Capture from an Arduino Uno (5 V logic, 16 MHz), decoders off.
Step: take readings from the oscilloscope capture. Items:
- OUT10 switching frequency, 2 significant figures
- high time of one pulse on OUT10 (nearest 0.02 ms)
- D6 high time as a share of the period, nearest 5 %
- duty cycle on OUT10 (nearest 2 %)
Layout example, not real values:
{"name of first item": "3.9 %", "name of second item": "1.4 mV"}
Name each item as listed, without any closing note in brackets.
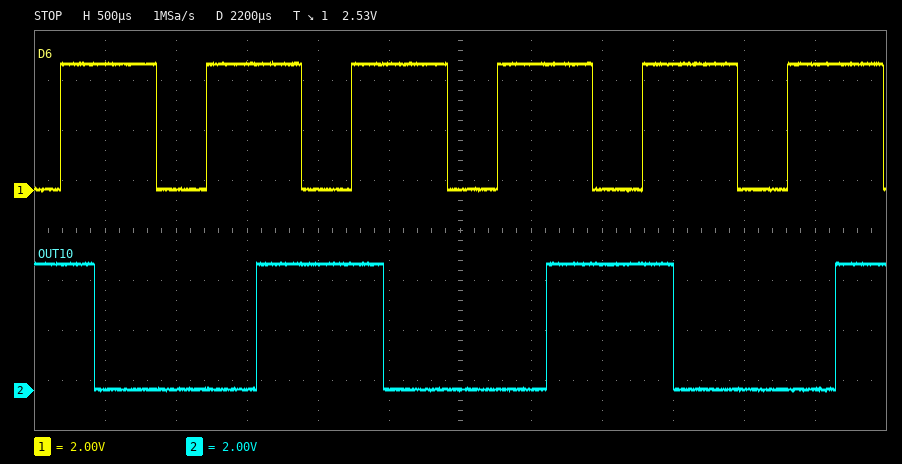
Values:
{"OUT10 switching frequency, 2 significant figures": "490 Hz", "high time of one pulse on OUT10": "0.90 ms", "D6 high time as a share of the period, nearest 5 %": "65 %", "duty cycle on OUT10": "44 %"}
